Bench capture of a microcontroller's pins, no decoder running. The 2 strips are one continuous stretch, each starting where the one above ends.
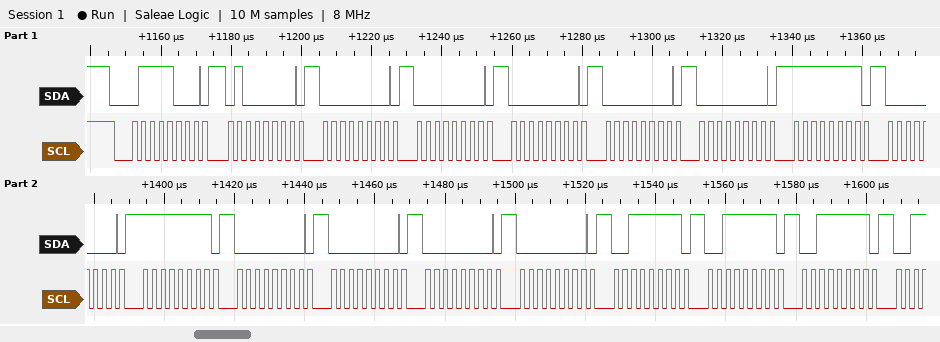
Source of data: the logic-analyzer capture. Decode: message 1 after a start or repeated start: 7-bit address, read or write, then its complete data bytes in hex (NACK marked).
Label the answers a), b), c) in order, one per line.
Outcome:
a) 0x3C write: 40 00 00 00 00 00 FF 00 FF 00 00 00 00 3F 3F 3F
